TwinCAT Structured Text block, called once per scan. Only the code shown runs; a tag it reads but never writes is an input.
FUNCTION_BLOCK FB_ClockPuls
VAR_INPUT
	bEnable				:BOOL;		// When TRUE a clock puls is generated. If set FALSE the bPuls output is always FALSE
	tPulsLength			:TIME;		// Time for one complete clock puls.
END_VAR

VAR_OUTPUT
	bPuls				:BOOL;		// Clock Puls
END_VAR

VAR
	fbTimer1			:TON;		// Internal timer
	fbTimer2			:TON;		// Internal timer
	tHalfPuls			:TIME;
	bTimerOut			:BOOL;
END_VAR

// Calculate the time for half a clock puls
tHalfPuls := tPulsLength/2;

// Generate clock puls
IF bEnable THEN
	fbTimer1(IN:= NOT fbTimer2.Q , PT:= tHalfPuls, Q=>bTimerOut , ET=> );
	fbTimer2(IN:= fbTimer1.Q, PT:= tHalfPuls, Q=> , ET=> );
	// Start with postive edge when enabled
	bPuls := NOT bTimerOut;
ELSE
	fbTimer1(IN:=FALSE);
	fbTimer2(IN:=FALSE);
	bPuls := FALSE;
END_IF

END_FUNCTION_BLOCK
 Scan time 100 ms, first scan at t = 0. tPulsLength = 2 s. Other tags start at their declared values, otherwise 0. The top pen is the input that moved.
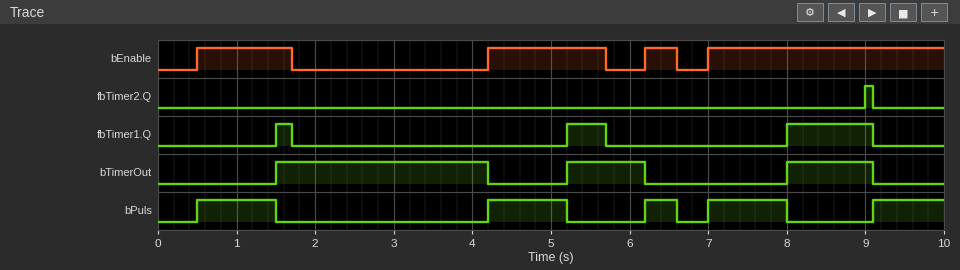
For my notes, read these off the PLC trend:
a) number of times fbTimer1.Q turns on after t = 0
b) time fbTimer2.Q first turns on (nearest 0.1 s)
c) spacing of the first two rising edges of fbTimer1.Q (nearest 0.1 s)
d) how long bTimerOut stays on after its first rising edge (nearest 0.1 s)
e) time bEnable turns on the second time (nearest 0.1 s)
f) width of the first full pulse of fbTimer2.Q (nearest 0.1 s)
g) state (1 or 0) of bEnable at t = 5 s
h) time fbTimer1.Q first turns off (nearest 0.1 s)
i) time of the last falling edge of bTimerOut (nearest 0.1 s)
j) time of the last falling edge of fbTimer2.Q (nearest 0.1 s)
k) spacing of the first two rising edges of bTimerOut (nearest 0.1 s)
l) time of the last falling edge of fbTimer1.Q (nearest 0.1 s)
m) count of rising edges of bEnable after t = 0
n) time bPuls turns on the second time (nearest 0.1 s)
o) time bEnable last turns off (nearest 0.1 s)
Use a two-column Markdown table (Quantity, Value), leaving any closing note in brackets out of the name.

| Quantity | Value |
|---|---|
| number of times fbTimer1.Q turns on after t = 0 | 3 |
| time fbTimer2.Q first turns on | 9.0 s |
| spacing of the first two rising edges of fbTimer1.Q | 3.7 s |
| how long bTimerOut stays on after its first rising edge | 2.7 s |
| time bEnable turns on the second time | 4.2 s |
| width of the first full pulse of fbTimer2.Q | 0.1 s |
| state (1 or 0) of bEnable at t = 5 s | 1 |
| time fbTimer1.Q first turns off | 1.7 s |
| time of the last falling edge of bTimerOut | 9.1 s |
| time of the last falling edge of fbTimer2.Q | 9.1 s |
| spacing of the first two rising edges of bTimerOut | 3.7 s |
| time of the last falling edge of fbTimer1.Q | 9.1 s |
| count of rising edges of bEnable after t = 0 | 4 |
| time bPuls turns on the second time | 4.2 s |
| time bEnable last turns off | 6.6 s |
